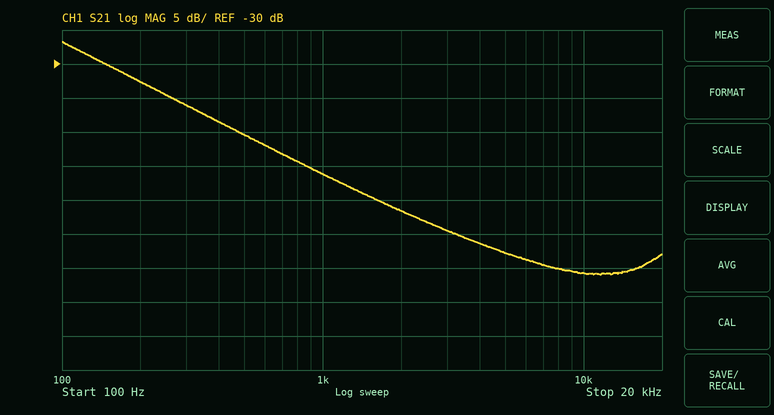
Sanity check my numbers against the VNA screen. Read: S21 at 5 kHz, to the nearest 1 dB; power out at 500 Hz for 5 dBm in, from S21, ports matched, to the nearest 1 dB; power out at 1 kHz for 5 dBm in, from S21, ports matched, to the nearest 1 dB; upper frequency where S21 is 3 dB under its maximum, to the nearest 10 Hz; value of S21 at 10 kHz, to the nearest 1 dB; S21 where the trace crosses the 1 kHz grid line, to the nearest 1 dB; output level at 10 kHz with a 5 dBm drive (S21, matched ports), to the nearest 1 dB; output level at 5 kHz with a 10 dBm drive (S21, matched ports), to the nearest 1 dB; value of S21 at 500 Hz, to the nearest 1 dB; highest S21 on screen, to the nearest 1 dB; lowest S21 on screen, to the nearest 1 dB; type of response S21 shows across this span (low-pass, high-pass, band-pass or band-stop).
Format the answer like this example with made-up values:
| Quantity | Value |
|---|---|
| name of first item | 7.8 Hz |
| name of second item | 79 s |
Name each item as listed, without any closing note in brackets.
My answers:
| Quantity | Value |
|---|---|
| S21 at 5 kHz, to the nearest 1 dB | -58 dB |
| power out at 500 Hz for 5 dBm in, from S21, ports matched, to the nearest 1 dB | -35 dBm |
| power out at 1 kHz for 5 dBm in, from S21, ports matched, to the nearest 1 dB | -41 dBm |
| upper frequency where S21 is 3 dB under its maximum, to the nearest 10 Hz | 140 Hz |
| value of S21 at 10 kHz, to the nearest 1 dB | -61 dB |
| S21 where the trace crosses the 1 kHz grid line, to the nearest 1 dB | -46 dB |
| output level at 10 kHz with a 5 dBm drive (S21, matched ports), to the nearest 1 dB | -56 dBm |
| output level at 5 kHz with a 10 dBm drive (S21, matched ports), to the nearest 1 dB | -48 dBm |
| value of S21 at 500 Hz, to the nearest 1 dB | -40 dB |
| highest S21 on screen, to the nearest 1 dB | -27 dB |
| lowest S21 on screen, to the nearest 1 dB | -61 dB |
| type of response S21 shows across this span | low-pass |
